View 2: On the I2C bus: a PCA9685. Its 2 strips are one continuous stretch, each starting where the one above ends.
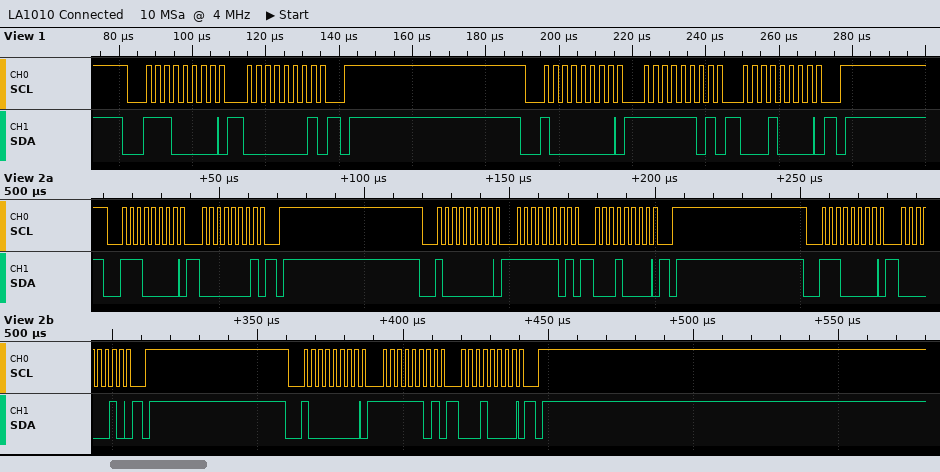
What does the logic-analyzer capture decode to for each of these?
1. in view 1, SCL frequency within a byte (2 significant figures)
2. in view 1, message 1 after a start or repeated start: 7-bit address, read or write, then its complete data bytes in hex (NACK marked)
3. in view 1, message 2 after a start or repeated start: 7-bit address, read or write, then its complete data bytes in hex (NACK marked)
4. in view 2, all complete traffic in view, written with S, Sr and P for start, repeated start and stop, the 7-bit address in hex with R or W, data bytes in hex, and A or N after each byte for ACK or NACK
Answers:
400 kHz
0x70 write: 01
0x40 write: FD 10
S 70W A 01 A P S 40W A FD A 10 A P S 70W A 02 A P S 40W A FD A 10 A P
